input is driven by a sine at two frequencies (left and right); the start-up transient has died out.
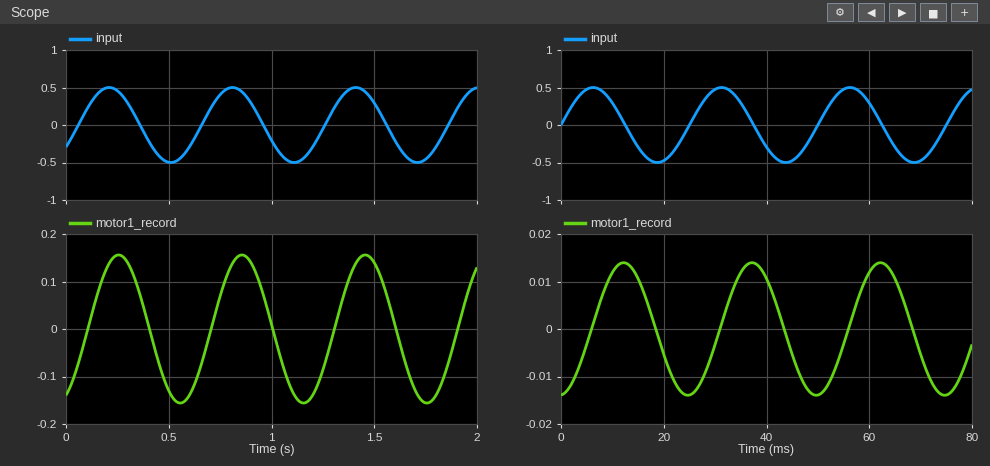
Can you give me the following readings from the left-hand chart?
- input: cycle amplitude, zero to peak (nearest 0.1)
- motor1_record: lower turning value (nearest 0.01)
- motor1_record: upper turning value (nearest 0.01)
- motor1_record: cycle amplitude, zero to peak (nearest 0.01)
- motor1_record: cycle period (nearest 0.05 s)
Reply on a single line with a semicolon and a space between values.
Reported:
0.5; -0.16; 0.16; 0.16; 0.60 s
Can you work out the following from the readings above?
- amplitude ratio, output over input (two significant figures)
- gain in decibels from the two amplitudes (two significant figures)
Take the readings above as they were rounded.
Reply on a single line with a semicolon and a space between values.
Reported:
0.32; -9.9 dB
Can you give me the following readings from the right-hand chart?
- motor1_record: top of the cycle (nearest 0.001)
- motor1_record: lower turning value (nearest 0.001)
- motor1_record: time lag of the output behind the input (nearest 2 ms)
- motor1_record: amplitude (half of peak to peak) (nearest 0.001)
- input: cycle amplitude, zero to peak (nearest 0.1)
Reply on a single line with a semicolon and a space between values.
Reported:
0.014; -0.014; 6 ms; 0.014; 0.5
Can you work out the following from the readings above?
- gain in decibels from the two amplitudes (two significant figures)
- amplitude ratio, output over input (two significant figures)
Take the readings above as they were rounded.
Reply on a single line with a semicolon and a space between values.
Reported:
-31 dB; 0.028
